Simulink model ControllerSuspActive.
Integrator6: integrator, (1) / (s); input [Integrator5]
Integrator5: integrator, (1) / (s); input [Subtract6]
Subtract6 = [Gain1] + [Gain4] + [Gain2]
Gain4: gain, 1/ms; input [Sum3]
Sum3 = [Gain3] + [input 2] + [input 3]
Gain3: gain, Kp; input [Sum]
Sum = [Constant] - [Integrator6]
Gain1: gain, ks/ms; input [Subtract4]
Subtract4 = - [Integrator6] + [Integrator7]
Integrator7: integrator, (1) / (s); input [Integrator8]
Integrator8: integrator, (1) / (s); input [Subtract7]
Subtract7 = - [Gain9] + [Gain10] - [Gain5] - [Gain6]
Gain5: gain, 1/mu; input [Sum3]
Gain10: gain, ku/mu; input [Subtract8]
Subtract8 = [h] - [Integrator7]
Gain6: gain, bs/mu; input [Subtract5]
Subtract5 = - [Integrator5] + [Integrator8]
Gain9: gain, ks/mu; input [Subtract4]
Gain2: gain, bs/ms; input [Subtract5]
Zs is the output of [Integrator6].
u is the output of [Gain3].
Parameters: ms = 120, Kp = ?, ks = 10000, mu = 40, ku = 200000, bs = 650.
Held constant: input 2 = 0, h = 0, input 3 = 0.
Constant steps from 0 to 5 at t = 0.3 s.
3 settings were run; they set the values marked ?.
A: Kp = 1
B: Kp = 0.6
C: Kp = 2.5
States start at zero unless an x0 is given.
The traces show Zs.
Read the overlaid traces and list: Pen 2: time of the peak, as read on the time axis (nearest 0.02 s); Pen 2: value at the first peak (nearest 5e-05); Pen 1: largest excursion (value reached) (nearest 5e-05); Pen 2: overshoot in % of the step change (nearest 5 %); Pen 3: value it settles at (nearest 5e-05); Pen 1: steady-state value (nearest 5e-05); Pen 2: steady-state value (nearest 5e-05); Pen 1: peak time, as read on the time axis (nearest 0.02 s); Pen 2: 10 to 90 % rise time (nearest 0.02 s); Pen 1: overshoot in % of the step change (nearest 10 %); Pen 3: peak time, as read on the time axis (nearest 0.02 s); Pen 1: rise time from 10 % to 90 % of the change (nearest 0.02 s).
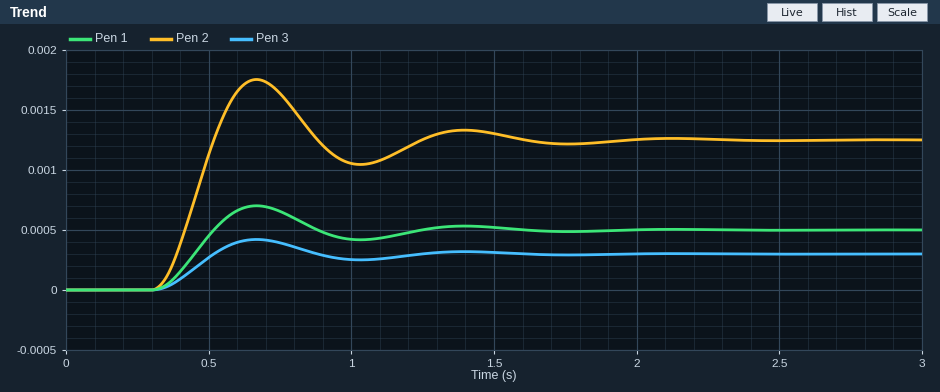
0.66 s
0.00175
0.00070
40 %
0.00030
0.00050
0.00125
0.66 s
0.14 s
40 %
0.66 s
0.14 s
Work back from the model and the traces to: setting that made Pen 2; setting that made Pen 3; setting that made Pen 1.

C
B
A
